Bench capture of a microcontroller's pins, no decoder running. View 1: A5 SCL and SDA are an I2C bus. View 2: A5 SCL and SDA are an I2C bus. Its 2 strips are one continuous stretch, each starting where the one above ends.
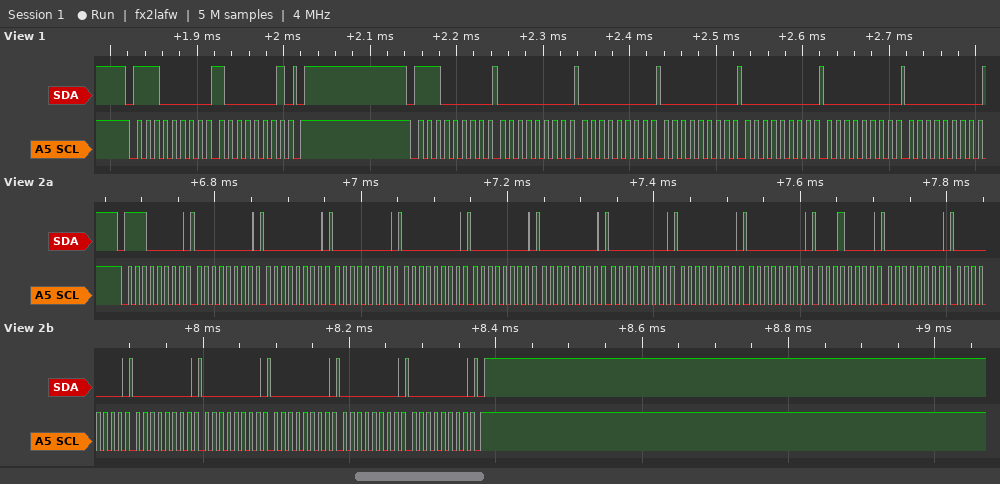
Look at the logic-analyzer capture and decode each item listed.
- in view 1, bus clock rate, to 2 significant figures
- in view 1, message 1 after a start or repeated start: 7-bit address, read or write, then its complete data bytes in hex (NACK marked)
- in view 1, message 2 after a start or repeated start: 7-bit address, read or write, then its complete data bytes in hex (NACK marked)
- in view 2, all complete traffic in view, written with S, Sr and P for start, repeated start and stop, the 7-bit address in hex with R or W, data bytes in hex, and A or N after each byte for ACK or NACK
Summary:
100 kHz
0x70 write: 81
0x70 write: 00 00 00 00 00 00
S 70W A 00 A 00 A 00 A 00 A 00 A 00 A 00 A 00 A 00 A 10 A 00 A 00 A 00 A 00 A 00 A 00 A 00 A P
